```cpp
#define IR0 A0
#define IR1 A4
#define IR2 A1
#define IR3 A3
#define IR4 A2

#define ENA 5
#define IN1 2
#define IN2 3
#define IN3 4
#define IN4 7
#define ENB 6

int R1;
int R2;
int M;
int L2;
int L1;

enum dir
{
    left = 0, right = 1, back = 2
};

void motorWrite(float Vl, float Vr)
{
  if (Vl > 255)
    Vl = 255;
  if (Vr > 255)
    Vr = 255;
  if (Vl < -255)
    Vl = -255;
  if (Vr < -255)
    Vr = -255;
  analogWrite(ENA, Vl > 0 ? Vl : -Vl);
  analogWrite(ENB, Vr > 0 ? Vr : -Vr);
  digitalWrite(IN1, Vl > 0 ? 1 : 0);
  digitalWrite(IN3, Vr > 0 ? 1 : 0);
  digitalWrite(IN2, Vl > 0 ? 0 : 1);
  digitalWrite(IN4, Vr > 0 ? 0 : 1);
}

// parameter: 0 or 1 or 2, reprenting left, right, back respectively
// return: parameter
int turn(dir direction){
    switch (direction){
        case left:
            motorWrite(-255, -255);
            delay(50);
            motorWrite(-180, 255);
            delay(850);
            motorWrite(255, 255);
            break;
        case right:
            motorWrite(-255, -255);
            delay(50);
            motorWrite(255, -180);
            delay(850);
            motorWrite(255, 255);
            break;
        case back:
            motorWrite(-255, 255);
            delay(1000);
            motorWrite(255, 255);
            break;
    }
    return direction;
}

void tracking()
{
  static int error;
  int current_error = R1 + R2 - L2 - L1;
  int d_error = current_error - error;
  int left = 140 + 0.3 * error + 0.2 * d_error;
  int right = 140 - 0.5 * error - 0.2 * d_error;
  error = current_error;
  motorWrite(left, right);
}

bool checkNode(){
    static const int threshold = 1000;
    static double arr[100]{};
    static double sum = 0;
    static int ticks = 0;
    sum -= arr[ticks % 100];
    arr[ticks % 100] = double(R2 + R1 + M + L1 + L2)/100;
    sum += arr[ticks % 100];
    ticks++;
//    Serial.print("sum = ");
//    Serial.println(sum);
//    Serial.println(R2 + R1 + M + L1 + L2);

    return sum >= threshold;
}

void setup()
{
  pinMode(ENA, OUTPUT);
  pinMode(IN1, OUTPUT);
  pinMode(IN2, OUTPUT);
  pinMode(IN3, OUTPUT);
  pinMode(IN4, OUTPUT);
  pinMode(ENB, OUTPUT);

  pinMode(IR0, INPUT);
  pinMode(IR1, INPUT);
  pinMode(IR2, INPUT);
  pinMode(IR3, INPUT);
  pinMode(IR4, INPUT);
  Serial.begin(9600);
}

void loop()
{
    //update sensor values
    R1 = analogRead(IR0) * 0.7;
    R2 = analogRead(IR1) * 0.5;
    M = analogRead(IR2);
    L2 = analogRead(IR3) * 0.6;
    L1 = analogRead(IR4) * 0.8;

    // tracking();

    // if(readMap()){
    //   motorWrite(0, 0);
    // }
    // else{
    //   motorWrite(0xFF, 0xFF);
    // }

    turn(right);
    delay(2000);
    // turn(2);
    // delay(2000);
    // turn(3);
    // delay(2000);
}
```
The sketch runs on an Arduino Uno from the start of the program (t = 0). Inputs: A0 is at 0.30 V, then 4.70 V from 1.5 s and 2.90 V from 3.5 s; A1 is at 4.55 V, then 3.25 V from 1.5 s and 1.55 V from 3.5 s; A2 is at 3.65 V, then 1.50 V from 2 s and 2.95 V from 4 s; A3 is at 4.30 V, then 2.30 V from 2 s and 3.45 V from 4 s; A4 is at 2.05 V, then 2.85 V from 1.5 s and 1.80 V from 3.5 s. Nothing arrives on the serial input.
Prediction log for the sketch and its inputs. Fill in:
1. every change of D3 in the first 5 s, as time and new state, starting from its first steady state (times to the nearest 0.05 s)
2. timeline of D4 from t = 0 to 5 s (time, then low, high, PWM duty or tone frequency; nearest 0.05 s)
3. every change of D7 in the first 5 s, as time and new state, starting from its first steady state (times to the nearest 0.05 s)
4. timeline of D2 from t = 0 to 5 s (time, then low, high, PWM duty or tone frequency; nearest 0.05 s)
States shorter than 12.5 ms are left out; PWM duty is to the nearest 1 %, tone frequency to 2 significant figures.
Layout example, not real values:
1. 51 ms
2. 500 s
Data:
1. 0 s high; 0.05 s low; 2.9 s high; 2.95 s low
2. 0 s low; 0.9 s high; 2.9 s low; 3.8 s high
3. 0 s high; 0.9 s low; 2.9 s high; 3.8 s low
4. 0 s low; 0.05 s high; 2.9 s low; 2.95 s high
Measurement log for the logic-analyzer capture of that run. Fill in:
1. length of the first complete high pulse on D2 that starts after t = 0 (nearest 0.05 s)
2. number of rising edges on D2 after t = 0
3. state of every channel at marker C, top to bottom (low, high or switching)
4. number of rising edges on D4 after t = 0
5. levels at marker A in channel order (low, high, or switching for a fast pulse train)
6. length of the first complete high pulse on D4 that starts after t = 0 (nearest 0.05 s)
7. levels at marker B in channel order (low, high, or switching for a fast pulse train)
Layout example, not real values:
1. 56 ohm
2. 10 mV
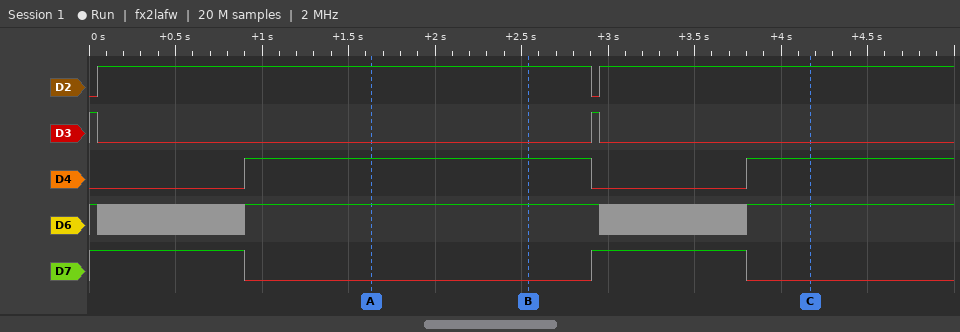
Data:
1. 2.85 s
2. 2
3. D2 high, D3 low, D4 high, D6 high, D7 low
4. 2
5. D2 high, D3 low, D4 high, D6 high, D7 low
6. 2.00 s
7. D2 high, D3 low, D4 high, D6 high, D7 low
